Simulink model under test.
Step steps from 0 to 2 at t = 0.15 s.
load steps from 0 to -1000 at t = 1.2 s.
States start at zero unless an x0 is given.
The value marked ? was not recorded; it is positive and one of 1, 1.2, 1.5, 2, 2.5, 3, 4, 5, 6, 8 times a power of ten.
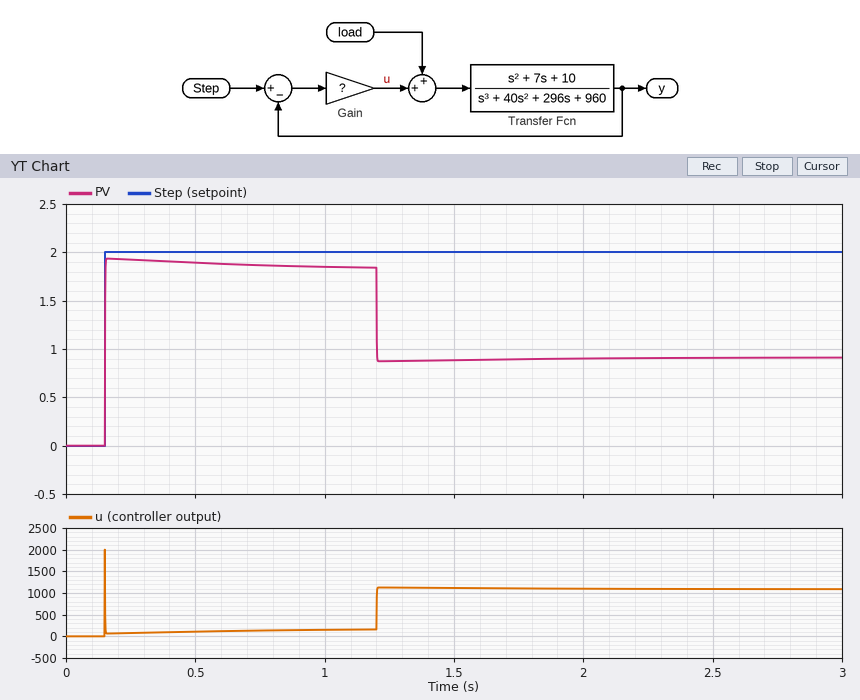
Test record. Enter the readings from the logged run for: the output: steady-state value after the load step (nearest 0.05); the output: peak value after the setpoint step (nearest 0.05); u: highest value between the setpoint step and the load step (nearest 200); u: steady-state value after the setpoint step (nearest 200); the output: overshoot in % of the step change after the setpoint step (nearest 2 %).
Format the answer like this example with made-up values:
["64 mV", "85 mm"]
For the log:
["0.90", "1.95", "2000", "200", "6 %"]
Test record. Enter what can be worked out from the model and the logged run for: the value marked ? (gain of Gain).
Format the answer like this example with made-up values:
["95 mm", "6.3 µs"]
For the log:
["1000"]
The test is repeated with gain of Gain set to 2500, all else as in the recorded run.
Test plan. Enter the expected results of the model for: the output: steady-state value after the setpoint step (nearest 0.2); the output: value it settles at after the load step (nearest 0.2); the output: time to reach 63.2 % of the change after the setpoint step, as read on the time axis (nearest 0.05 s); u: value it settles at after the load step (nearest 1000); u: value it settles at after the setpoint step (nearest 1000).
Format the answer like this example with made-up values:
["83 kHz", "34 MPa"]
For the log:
["2.0", "1.6", "0.15 s", "1000", "0"]
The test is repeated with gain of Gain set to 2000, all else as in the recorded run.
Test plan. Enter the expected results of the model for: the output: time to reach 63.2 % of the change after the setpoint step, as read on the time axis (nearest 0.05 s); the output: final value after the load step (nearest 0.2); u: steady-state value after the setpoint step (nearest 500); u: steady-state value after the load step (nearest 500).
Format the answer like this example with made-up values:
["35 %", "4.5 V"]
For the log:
["0.15 s", "1.4", "0", "1000"]
